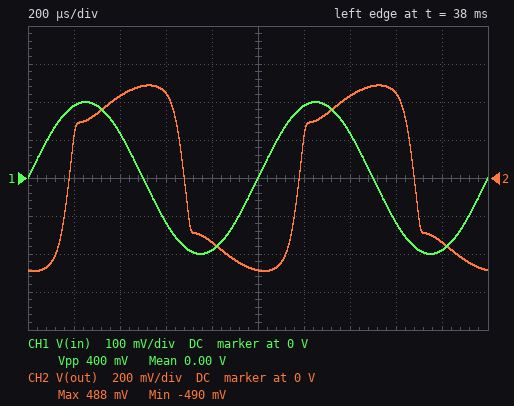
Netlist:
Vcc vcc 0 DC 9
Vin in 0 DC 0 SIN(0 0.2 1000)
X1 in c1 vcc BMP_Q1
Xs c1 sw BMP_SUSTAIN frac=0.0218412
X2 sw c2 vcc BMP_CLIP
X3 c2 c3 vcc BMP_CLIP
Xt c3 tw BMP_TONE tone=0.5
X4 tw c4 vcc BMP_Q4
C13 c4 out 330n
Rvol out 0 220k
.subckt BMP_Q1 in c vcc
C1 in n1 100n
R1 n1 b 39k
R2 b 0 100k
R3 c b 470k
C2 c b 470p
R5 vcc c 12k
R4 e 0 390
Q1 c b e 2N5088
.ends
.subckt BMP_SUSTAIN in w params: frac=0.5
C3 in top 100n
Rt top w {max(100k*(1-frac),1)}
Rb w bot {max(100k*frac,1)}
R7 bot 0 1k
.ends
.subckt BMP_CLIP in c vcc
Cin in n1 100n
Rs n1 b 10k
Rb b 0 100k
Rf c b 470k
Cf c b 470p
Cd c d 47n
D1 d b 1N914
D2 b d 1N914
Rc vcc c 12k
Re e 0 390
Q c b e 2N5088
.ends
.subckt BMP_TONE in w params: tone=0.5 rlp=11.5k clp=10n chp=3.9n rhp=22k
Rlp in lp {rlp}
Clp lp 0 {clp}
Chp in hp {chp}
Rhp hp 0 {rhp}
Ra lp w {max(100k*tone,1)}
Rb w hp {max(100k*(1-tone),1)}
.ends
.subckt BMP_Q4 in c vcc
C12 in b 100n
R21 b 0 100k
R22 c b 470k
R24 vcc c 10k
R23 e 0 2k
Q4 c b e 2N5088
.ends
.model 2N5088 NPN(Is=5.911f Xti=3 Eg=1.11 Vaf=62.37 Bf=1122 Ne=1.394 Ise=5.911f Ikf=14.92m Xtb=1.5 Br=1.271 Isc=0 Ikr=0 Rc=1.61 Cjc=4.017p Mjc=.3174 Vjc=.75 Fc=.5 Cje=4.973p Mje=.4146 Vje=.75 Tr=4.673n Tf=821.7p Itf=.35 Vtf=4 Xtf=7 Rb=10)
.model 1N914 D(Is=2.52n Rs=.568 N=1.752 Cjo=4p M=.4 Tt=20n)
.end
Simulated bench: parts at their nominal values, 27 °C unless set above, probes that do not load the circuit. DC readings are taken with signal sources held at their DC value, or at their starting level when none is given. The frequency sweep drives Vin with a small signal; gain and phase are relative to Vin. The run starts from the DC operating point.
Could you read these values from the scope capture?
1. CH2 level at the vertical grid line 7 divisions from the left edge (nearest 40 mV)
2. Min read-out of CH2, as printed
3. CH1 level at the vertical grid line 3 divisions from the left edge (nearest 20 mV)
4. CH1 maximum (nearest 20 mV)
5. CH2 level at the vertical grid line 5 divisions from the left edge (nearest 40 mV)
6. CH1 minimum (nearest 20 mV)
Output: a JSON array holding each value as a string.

["440 mV", "-490 mV", "-120 mV", "200 mV", "-480 mV", "-200 mV"]
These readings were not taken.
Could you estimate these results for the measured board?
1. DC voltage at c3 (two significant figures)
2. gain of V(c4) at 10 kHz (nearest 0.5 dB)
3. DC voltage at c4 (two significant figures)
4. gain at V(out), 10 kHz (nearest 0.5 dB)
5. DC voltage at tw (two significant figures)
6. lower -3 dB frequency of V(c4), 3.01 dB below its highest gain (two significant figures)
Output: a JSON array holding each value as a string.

["4.6 V", "-14.5 dB", "6.5 V", "-14.5 dB", "2.5 V", "74 Hz"]
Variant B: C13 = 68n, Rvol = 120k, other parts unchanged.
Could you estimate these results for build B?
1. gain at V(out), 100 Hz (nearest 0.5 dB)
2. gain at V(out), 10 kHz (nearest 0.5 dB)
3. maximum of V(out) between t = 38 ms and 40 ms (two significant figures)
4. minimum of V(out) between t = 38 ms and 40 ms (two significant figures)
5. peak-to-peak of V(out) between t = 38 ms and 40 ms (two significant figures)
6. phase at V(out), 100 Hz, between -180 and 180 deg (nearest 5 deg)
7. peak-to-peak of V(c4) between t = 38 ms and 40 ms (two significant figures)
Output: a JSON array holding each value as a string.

["28.0 dB", "-15.0 dB", "470 mV", "-470 mV", "940 mV", "85 deg", "950 mV"]
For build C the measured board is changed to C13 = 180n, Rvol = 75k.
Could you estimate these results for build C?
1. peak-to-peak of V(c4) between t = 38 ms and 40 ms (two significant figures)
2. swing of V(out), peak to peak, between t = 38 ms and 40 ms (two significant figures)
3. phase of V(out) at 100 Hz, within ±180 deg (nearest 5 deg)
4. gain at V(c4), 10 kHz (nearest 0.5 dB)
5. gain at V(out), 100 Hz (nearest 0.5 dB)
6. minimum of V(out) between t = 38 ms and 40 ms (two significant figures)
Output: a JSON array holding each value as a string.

["920 mV", "910 mV", "80 deg", "-15.0 dB", "28.0 dB", "-460 mV"]
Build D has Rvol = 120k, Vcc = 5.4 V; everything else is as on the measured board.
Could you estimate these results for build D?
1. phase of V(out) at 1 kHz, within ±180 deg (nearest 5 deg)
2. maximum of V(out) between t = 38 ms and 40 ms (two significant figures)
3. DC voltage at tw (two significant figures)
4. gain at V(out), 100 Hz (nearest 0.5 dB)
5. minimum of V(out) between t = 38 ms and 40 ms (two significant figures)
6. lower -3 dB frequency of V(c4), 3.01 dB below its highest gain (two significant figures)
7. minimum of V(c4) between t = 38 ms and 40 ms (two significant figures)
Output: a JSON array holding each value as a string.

["-90 deg", "390 mV", "2.0 V", "23.5 dB", "-400 mV", "69 Hz", "4.1 V"]
